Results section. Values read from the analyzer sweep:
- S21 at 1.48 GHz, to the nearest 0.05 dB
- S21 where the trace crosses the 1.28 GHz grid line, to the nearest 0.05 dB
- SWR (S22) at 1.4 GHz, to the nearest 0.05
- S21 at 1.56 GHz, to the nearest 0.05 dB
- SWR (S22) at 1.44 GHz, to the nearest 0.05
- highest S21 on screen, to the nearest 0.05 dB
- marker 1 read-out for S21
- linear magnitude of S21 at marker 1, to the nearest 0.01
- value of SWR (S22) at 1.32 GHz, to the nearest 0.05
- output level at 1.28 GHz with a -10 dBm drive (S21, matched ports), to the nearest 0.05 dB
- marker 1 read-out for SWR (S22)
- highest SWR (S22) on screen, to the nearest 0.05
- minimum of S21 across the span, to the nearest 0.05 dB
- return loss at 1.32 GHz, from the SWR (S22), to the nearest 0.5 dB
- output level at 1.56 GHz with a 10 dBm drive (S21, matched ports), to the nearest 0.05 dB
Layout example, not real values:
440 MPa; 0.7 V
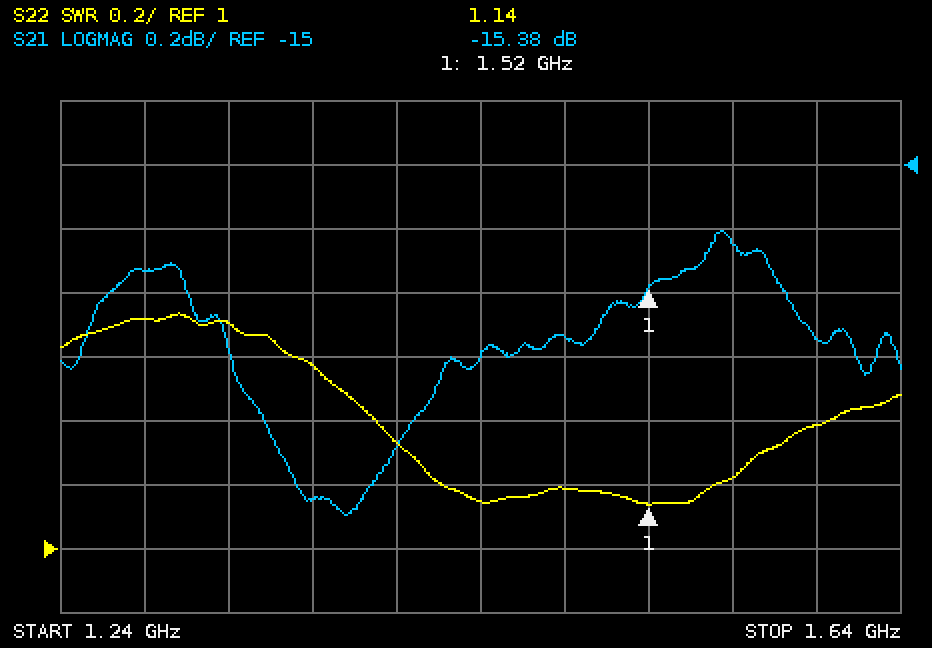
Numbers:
-15.55 dB; -15.35 dB; 1.35; -15.25 dB; 1.15; -15.20 dB; -15.38 dB; 0.17; 1.70; -25.35 dBm; 1.14; 1.75; -16.10 dB; 11.5 dB; -5.25 dBm
